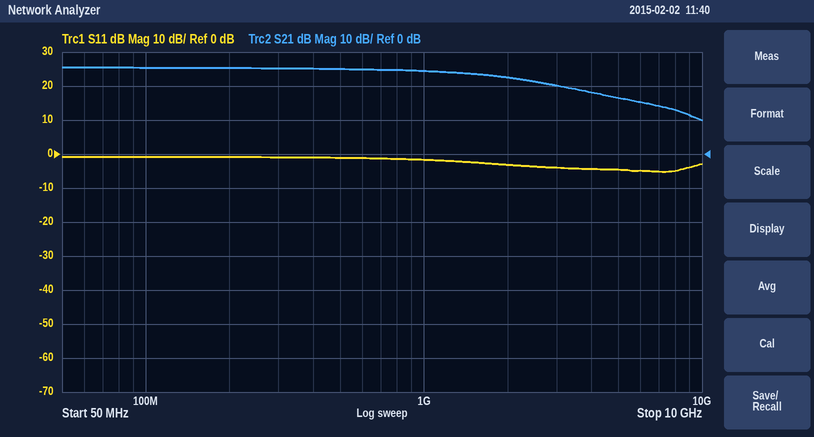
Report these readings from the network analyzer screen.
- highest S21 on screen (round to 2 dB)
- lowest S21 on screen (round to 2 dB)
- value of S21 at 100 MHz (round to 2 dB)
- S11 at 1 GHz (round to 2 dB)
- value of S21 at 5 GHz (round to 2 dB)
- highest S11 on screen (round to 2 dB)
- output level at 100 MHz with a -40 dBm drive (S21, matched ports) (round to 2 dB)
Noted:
26 dB
10 dB
26 dB
-2 dB
16 dB
0 dB
-14 dBm
